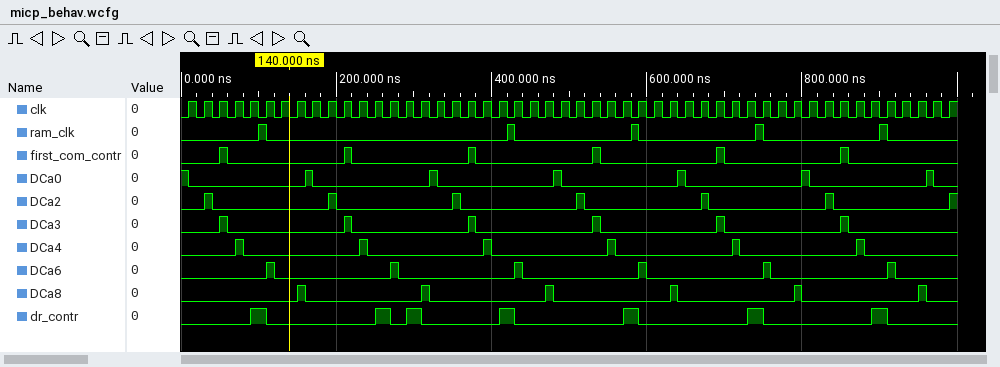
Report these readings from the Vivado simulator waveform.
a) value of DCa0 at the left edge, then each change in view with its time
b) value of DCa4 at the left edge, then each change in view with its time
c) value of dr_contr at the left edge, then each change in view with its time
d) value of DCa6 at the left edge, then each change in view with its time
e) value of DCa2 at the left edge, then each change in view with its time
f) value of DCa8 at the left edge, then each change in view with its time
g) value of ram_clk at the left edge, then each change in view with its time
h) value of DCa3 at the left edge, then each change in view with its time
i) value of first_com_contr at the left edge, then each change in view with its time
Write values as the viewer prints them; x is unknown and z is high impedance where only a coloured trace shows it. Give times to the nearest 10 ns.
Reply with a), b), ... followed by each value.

a) 1, 0 at 10 ns, 1 at 160 ns, 0 at 170 ns, 1 at 320 ns, 0 at 330 ns, 1 at 480 ns, 0 at 490 ns, 1 at 640 ns, 0 at 650 ns, 1 at 800 ns, 0 at 810 ns, 1 at 960 ns, 0 at 970 ns
b) 0, 1 at 70 ns, 0 at 80 ns, 1 at 230 ns, 0 at 240 ns, 1 at 390 ns, 0 at 400 ns, 1 at 550 ns, 0 at 560 ns, 1 at 710 ns, 0 at 720 ns, 1 at 870 ns, 0 at 880 ns
c) 0, 1 at 90 ns, 0 at 110 ns, 1 at 250 ns, 0 at 270 ns, 1 at 290 ns, 0 at 310 ns, 1 at 410 ns, 0 at 430 ns, 1 at 570 ns, 0 at 590 ns, 1 at 730 ns, 0 at 750 ns, 1 at 890 ns, 0 at 910 ns
d) 0, 1 at 110 ns, 0 at 120 ns, 1 at 270 ns, 0 at 280 ns, 1 at 430 ns, 0 at 440 ns, 1 at 590 ns, 0 at 600 ns, 1 at 750 ns, 0 at 760 ns, 1 at 910 ns, 0 at 920 ns
e) 0, 1 at 30 ns, 0 at 40 ns, 1 at 190 ns, 0 at 200 ns, 1 at 350 ns, 0 at 360 ns, 1 at 510 ns, 0 at 520 ns, 1 at 670 ns, 0 at 680 ns, 1 at 830 ns, 0 at 840 ns, 1 at 990 ns
f) 0, 1 at 150 ns, 0 at 160 ns, 1 at 310 ns, 0 at 320 ns, 1 at 470 ns, 0 at 480 ns, 1 at 630 ns, 0 at 640 ns, 1 at 790 ns, 0 at 800 ns, 1 at 950 ns, 0 at 960 ns
g) 0, 1 at 100 ns, 0 at 110 ns, 1 at 420 ns, 0 at 430 ns, 1 at 580 ns, 0 at 590 ns, 1 at 740 ns, 0 at 750 ns, 1 at 900 ns, 0 at 910 ns
h) 0, 1 at 50 ns, 0 at 60 ns, 1 at 210 ns, 0 at 220 ns, 1 at 370 ns, 0 at 380 ns, 1 at 530 ns, 0 at 540 ns, 1 at 690 ns, 0 at 700 ns, 1 at 850 ns, 0 at 860 ns
i) 0, 1 at 50 ns, 0 at 60 ns, 1 at 210 ns, 0 at 220 ns, 1 at 370 ns, 0 at 380 ns, 1 at 530 ns, 0 at 540 ns, 1 at 690 ns, 0 at 700 ns, 1 at 850 ns, 0 at 860 ns
